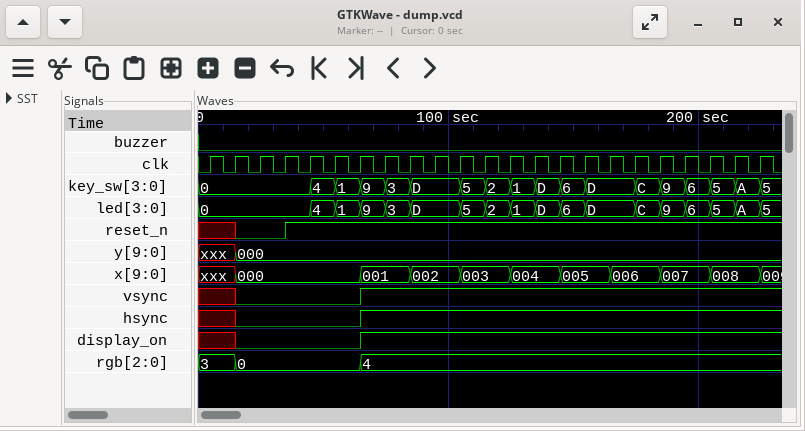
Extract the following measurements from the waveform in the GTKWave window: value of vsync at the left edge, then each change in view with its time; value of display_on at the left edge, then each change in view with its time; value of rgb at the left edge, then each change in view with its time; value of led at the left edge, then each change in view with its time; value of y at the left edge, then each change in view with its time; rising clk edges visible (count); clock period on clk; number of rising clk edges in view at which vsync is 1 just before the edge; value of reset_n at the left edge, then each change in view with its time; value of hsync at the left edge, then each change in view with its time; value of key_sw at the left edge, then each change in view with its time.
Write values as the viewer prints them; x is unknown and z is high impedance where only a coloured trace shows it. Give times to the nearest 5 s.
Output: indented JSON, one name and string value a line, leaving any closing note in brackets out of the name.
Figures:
{
  "value of vsync at the left edge, then each change in view with its time": "x, 0 at 15 s, 1 at 65 s",
  "value of display_on at the left edge, then each change in view with its time": "x, 0 at 15 s, 1 at 65 s",
  "value of rgb at the left edge, then each change in view with its time": "3, 0 at 15 s, 4 at 65 s",
  "value of led at the left edge, then each change in view with its time": "0, 4 at 45 s, 1 at 55 s, 9 at 65 s, 3 at 75 s, D at 85 s, 5 at 105 s, 2 at 115 s, 1 at 125 s, D at 135 s, 6 at 145 s, D at 155 s, C at 175 s, 9 at 185 s, 6 at 195 s, 5 at 205 s, A at 215 s, 5 at 225 s",
  "value of y at the left edge, then each change in view with its time": "xxx, 000 at 15 s",
  "rising clk edges visible": "23",
  "clock period on clk": "10 s",
  "number of rising clk edges in view at which vsync is 1 just before the edge": "16",
  "value of reset_n at the left edge, then each change in view with its time": "x, 0 at 15 s, 1 at 35 s",
  "value of hsync at the left edge, then each change in view with its time": "x, 0 at 15 s, 1 at 65 s",
  "value of key_sw at the left edge, then each change in view with its time": "0, 4 at 45 s, 1 at 55 s, 9 at 65 s, 3 at 75 s, D at 85 s, 5 at 105 s, 2 at 115 s, 1 at 125 s, D at 135 s, 6 at 145 s, D at 155 s, C at 175 s, 9 at 185 s, 6 at 195 s, 5 at 205 s, A at 215 s, 5 at 225 s"
}
